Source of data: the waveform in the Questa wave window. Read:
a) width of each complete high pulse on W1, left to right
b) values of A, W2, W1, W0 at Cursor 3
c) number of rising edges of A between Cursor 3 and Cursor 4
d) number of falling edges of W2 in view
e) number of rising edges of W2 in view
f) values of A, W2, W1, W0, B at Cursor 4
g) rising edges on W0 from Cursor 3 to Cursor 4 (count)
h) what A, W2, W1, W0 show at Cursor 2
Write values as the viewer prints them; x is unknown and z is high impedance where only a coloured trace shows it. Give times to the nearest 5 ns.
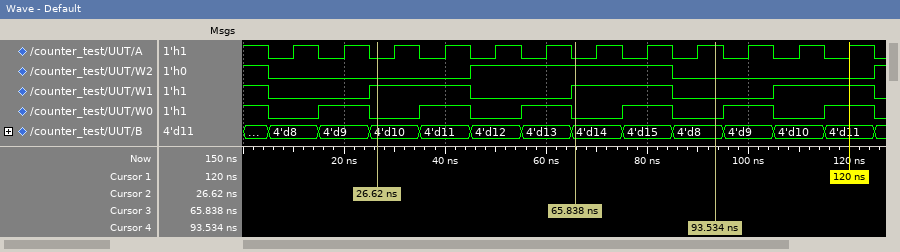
20 ns, 20 ns, 20 ns
A=0, W2=1, W1=1, W0=0
3
2
2
A=1, W2=0, W1=0, W0=0, B=4'd8
1
A=0, W2=0, W1=1, W0=0
